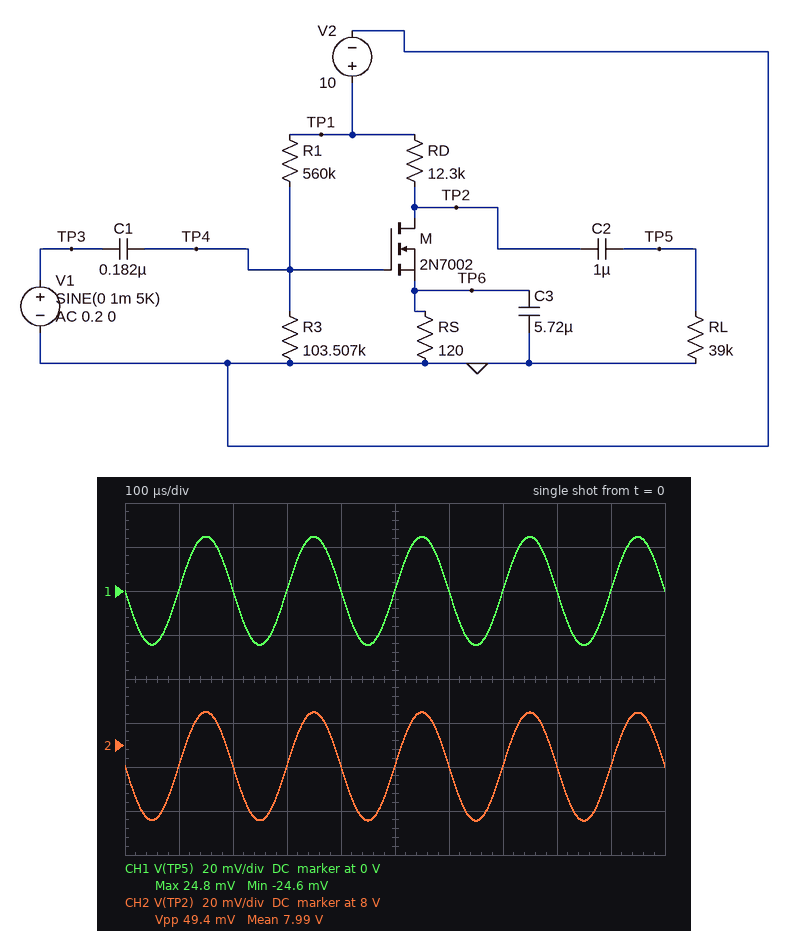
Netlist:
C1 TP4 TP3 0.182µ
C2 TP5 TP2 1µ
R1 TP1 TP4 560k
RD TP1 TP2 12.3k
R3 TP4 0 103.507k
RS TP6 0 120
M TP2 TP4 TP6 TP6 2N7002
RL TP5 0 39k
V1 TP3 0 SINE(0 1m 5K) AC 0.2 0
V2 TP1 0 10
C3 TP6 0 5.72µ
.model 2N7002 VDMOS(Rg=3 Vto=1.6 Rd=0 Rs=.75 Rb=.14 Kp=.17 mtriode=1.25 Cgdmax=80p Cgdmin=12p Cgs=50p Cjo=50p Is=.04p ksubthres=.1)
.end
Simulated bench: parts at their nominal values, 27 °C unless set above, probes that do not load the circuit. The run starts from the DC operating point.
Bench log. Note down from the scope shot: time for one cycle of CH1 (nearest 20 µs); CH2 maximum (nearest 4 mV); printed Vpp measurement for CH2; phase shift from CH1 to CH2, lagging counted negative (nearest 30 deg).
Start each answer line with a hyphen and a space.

- 200 µs
- 8.016 V
- 49.4 mV
- 0 deg
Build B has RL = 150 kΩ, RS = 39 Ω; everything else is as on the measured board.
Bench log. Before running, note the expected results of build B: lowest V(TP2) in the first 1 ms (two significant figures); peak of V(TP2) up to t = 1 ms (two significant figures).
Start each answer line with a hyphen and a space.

- 7.5 V
- 7.6 V
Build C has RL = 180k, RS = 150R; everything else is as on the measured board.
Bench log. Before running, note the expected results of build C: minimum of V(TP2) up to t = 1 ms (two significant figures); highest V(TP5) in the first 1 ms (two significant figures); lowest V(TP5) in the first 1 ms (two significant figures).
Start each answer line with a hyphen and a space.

- 8.1 V
- 29 mV
- -29 mV
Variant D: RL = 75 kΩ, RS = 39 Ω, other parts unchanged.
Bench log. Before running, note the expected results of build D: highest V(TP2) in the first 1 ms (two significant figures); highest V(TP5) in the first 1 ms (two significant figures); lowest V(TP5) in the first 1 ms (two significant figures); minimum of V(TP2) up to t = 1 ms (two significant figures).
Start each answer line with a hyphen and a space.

- 7.6 V
- 33 mV
- -33 mV
- 7.5 V
